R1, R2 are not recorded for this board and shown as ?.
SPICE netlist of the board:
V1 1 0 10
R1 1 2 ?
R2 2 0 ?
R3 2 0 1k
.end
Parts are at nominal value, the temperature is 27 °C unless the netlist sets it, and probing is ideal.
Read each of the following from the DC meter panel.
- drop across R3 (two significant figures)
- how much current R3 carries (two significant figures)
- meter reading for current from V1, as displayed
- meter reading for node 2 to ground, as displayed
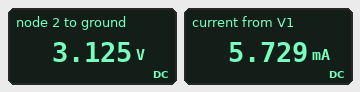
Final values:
3.1 V
3.1 mA
5.729 mA
3.125 V
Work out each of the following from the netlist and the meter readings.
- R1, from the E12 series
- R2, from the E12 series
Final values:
1.2 kΩ
1.2 kΩ
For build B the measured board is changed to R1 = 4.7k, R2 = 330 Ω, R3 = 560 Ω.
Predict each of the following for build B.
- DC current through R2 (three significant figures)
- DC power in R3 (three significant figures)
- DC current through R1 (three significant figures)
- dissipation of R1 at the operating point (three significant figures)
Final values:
1.28 mA
320 µW
2.04 mA
19.5 mW
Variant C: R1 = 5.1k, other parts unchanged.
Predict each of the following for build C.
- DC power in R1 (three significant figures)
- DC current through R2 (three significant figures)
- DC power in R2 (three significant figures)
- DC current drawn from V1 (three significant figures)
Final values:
16.0 mW
805 µA
778 µW
1.77 mA
